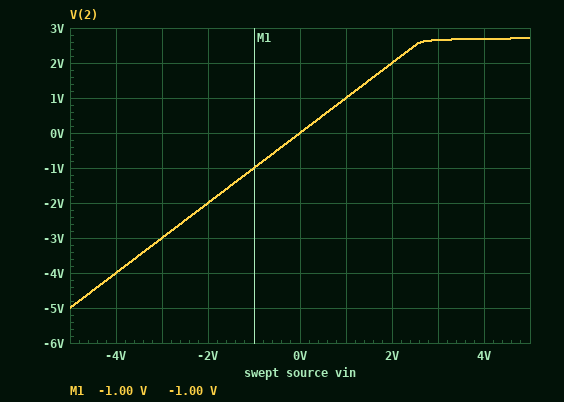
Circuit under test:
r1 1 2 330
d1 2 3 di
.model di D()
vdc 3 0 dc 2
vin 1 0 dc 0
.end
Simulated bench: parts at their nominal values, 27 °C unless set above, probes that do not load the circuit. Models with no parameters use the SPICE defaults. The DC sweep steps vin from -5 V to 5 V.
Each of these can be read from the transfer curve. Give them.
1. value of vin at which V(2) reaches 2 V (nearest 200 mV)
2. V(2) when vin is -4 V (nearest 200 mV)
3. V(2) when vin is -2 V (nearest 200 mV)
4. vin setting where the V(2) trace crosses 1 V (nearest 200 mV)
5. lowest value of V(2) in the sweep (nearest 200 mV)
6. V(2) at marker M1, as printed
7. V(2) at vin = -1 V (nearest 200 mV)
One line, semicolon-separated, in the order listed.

2.0 V; -4.0 V; -2.0 V; 1.0 V; -5.0 V; -1.00 V; -1.0 V
